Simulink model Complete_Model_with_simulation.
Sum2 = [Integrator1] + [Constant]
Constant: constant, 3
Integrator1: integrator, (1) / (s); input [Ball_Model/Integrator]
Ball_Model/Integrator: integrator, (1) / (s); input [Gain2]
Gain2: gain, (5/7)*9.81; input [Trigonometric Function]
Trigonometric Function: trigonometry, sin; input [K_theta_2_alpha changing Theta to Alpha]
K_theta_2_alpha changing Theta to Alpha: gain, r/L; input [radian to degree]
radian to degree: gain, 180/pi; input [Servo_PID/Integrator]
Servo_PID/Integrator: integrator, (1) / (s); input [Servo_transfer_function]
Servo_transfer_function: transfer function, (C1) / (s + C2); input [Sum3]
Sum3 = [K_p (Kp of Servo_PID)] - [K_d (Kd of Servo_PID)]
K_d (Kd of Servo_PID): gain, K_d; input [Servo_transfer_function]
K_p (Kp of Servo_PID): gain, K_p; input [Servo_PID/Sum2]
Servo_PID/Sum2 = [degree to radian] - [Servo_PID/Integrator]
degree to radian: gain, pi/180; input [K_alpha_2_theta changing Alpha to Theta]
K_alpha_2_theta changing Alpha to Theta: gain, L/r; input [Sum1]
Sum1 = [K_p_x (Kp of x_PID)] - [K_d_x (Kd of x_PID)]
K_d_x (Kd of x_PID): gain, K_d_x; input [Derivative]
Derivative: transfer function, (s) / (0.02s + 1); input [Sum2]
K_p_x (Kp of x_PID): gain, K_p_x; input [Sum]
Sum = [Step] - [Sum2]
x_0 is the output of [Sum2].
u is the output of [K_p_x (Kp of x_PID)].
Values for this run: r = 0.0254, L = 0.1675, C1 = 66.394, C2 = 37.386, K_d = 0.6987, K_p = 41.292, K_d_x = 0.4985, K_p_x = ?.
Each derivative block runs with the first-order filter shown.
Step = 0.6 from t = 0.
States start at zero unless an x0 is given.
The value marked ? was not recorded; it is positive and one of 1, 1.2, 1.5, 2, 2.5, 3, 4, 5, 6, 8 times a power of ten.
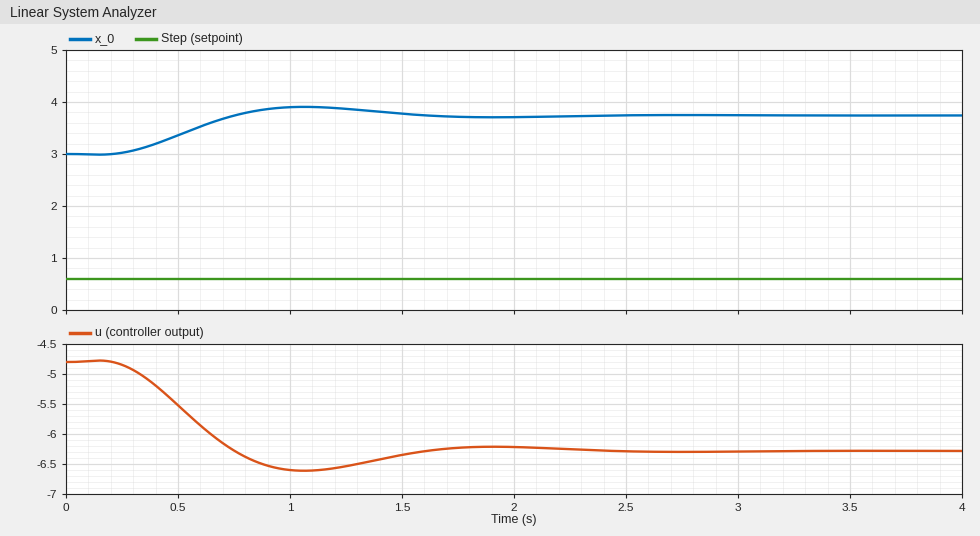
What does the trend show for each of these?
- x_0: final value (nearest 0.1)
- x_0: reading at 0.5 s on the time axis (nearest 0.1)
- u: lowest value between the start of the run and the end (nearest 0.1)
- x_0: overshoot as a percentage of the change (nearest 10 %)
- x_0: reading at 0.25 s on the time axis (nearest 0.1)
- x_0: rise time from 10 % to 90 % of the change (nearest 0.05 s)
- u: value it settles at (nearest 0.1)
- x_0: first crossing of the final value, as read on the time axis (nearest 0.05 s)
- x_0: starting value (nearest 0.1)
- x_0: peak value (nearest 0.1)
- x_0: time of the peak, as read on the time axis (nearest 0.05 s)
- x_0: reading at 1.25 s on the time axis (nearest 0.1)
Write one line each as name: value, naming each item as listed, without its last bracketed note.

x_0: final value: 3.7
x_0: reading at 0.5 s on the time axis: 3.4
u: lowest value between the start of the run and the end: -6.6
x_0: overshoot as a percentage of the change: 20 %
x_0: reading at 0.25 s on the time axis: 3.0
x_0: rise time from 10 % to 90 % of the change: 0.40 s
u: value it settles at: -6.3
x_0: first crossing of the final value, as read on the time axis: 0.75 s
x_0: starting value: 3.0
x_0: peak value: 3.9
x_0: time of the peak, as read on the time axis: 1.05 s
x_0: reading at 1.25 s on the time axis: 3.9
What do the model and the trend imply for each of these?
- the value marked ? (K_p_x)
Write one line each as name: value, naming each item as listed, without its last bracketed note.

the value marked ?: 2
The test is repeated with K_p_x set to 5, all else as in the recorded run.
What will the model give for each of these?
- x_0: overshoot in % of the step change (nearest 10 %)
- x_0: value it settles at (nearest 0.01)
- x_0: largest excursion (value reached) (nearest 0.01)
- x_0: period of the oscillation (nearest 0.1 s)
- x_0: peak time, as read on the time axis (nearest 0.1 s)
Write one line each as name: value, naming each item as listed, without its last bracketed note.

x_0: overshoot in % of the step change: 60 %
x_0: value it settles at: 3.11
x_0: largest excursion (value reached): 3.18
x_0: period of the oscillation: 1.0 s
x_0: peak time, as read on the time axis: 0.7 s
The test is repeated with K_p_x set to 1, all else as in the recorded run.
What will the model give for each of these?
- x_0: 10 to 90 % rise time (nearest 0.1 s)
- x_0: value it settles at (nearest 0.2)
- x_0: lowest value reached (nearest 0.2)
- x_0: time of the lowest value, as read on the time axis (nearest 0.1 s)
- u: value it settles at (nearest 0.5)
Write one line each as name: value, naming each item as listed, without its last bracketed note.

x_0: 10 to 90 % rise time: 0.8 s
x_0: value it settles at: 0.6
x_0: lowest value reached: 0.4
x_0: time of the lowest value, as read on the time axis: 1.8 s
u: value it settles at: 0.0
